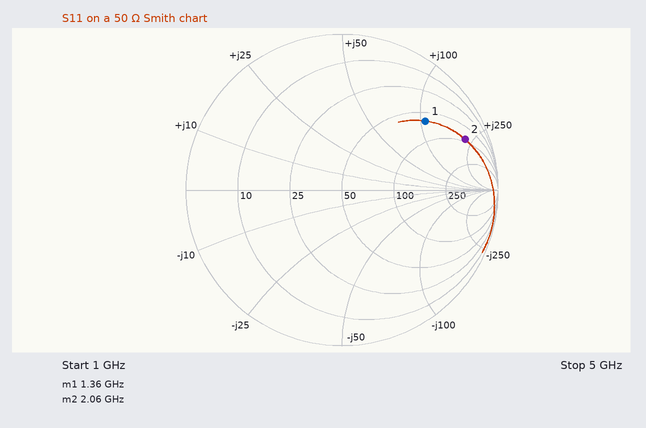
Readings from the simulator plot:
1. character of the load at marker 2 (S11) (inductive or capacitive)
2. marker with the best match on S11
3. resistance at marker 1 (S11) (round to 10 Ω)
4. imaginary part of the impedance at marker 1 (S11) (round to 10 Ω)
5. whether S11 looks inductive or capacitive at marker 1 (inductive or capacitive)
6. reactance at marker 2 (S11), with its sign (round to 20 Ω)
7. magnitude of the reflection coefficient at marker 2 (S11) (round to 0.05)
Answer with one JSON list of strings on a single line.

["inductive", "marker 1", "60 Ω", "+110 Ω", "inductive", "+220 Ω", "0.85"]
